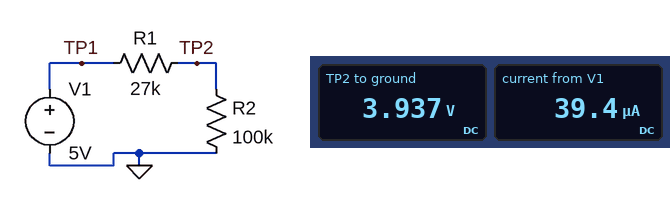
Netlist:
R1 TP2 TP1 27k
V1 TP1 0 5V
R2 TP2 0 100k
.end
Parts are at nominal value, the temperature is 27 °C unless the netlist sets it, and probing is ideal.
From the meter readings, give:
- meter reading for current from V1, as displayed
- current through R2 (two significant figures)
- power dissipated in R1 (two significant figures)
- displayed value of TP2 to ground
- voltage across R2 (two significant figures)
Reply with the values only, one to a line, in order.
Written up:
39.4 µA
39 µA
42 µW
3.937 V
3.9 V
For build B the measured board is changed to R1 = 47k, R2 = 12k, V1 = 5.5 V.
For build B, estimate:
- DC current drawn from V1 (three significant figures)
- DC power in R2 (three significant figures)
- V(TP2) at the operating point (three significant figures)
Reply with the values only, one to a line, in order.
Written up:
93.2 µA
104 µW
1.12 V
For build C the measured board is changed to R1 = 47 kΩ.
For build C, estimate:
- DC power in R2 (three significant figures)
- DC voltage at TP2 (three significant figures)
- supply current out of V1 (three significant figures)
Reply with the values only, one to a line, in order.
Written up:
116 µW
3.40 V
34.0 µA
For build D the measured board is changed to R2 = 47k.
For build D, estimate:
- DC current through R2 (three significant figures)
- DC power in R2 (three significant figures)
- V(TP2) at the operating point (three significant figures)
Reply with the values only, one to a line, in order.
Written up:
67.6 µA
215 µW
3.18 V
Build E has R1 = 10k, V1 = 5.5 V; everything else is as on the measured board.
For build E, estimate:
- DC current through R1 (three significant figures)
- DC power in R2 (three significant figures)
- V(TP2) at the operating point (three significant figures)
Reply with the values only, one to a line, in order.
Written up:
50.0 µA
250 µW
5.00 V
